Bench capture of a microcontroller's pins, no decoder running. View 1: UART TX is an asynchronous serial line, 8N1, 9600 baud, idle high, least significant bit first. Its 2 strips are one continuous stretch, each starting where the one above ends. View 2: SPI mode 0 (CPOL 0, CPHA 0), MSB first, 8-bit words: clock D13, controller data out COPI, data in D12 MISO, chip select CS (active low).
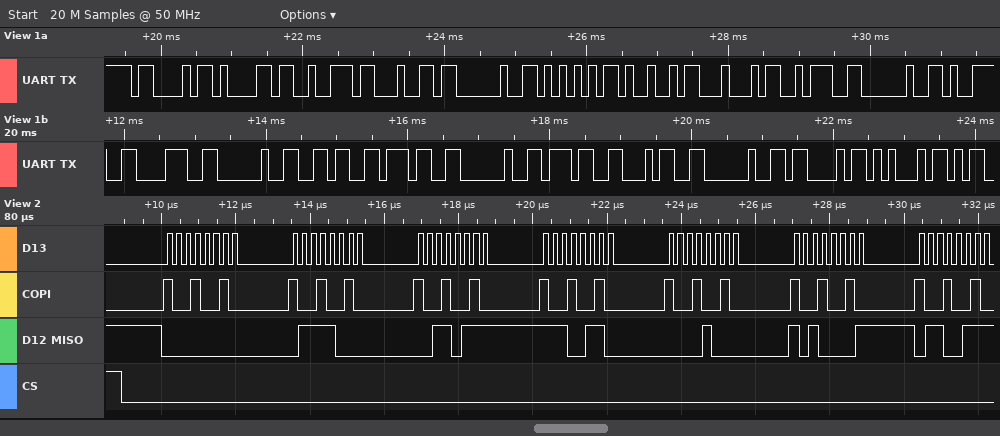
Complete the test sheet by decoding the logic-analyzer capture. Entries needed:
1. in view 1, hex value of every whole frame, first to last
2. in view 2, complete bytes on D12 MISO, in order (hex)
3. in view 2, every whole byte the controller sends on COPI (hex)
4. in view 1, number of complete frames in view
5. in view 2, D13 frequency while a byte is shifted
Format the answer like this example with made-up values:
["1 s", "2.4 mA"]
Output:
["43 61 72 64 20 55 49 44 3A 20 39 38 20 36 37 20 37 34 20 43 45", "00 78 37 E6 08 A1 67", "92 92 92 92 92 92 92", "21", "4 MHz"]
